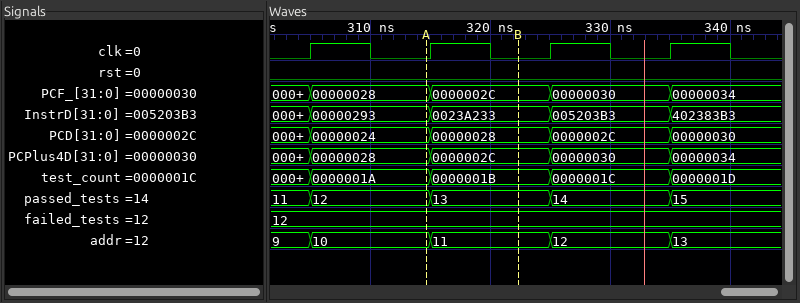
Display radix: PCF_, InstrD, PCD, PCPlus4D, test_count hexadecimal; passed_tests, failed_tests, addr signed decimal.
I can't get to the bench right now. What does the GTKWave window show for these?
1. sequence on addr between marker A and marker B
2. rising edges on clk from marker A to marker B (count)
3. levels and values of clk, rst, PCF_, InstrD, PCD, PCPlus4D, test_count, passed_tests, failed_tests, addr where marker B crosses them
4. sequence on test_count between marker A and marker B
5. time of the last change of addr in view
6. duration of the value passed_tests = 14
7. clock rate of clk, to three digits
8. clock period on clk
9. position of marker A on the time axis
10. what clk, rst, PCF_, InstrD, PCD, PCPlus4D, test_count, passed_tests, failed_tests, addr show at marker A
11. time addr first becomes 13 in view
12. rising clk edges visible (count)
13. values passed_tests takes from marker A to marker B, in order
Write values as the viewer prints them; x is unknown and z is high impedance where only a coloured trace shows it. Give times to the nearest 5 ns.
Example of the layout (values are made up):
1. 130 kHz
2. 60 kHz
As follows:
1. 10, 11
2. 1
3. clk=0, rst=0, PCF_=0000002C, InstrD=0023A233, PCD=00000028, PCPlus4D=0000002C, test_count=0000001B, passed_tests=13, failed_tests=12, addr=11
4. 0000001A, 0000001B
5. 335 ns
6. 10 ns
7. 100 MHz
8. 10 ns
9. 315 ns
10. clk=0, rst=0, PCF_=00000028, InstrD=00000293, PCD=00000024, PCPlus4D=00000028, test_count=0000001A, passed_tests=12, failed_tests=12, addr=10
11. 335 ns
12. 4
13. 12, 13
